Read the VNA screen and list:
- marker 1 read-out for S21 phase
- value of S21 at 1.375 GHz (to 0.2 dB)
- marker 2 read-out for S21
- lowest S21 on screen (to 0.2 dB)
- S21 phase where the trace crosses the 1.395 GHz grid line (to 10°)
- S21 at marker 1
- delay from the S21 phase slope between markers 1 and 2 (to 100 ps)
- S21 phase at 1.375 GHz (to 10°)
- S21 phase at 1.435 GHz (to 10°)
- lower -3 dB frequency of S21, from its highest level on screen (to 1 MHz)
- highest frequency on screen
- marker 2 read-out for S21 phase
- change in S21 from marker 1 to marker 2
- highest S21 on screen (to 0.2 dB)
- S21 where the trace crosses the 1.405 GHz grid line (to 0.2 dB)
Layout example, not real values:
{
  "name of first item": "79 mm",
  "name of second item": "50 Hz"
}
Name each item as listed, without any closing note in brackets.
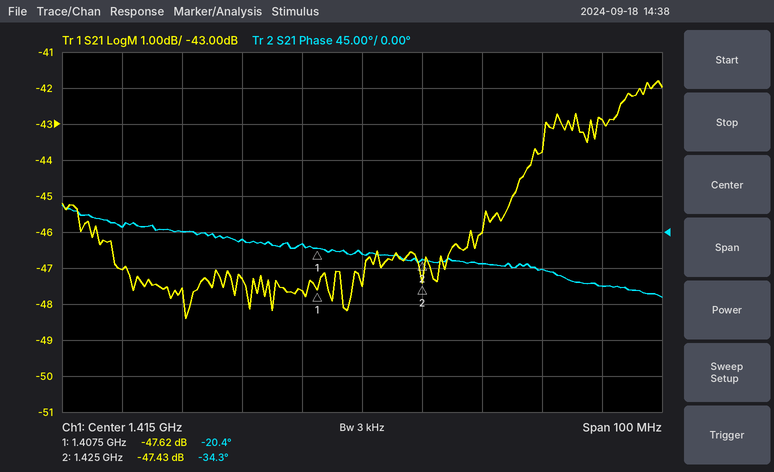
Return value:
{
  "marker 1 read-out for S21 phase": "-20.4°",
  "value of S21 at 1.375 GHz": "-47.0 dB",
  "marker 2 read-out for S21": "-47.43 dB",
  "lowest S21 on screen": "-48.4 dB",
  "S21 phase where the trace crosses the 1.395 GHz grid line": "-10°",
  "S21 at marker 1": "-47.62 dB",
  "delay from the S21 phase slope between markers 1 and 2": "2.2 ns",
  "S21 phase at 1.375 GHz": "10°",
  "S21 phase at 1.435 GHz": "-40°",
  "lower -3 dB frequency of S21, from its highest level on screen": "1.441 GHz",
  "highest frequency on screen": "1.465 GHz",
  "marker 2 read-out for S21 phase": "-34.3°",
  "change in S21 from marker 1 to marker 2": "0.19 dB",
  "highest S21 on screen": "-41.8 dB",
  "S21 where the trace crosses the 1.405 GHz grid line": "-47.6 dB"
}
